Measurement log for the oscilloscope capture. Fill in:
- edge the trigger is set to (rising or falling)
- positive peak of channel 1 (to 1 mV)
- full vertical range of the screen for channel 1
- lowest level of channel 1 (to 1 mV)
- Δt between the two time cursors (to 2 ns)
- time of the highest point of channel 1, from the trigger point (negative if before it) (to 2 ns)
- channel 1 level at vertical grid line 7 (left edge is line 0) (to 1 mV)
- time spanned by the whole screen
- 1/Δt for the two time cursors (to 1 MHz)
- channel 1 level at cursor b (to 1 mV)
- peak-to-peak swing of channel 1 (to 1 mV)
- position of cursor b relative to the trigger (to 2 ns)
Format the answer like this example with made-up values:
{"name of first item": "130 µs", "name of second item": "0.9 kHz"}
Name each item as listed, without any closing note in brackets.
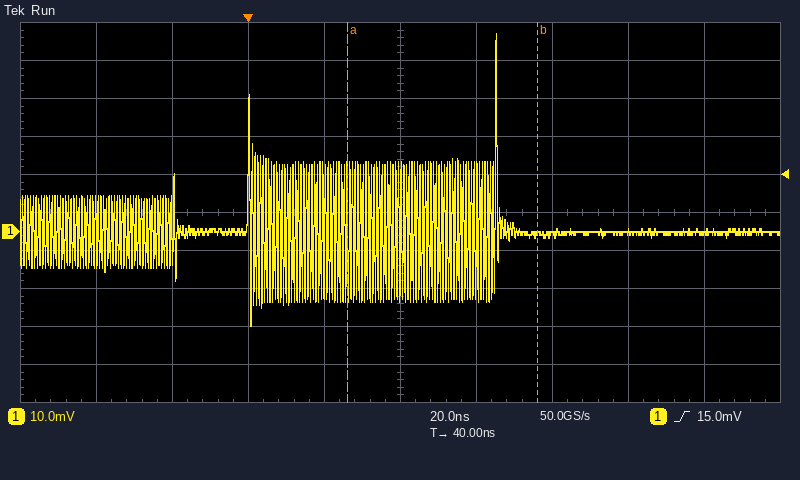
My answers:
{"edge the trigger is set to": "rising", "positive peak of channel 1": "52 mV", "full vertical range of the screen for channel 1": "100 mV", "lowest level of channel 1": "-25 mV", "Δt between the two time cursors": "50 ns", "time of the highest point of channel 1, from the trigger point (negative if before it)": "+66 ns", "channel 1 level at vertical grid line 7 (left edge is line 0)": "-1 mV", "time spanned by the whole screen": "200 ns", "1/Δt for the two time cursors": "20 MHz", "channel 1 level at cursor b": "-1 mV", "peak-to-peak swing of channel 1": "77 mV", "position of cursor b relative to the trigger": "+76 ns"}
